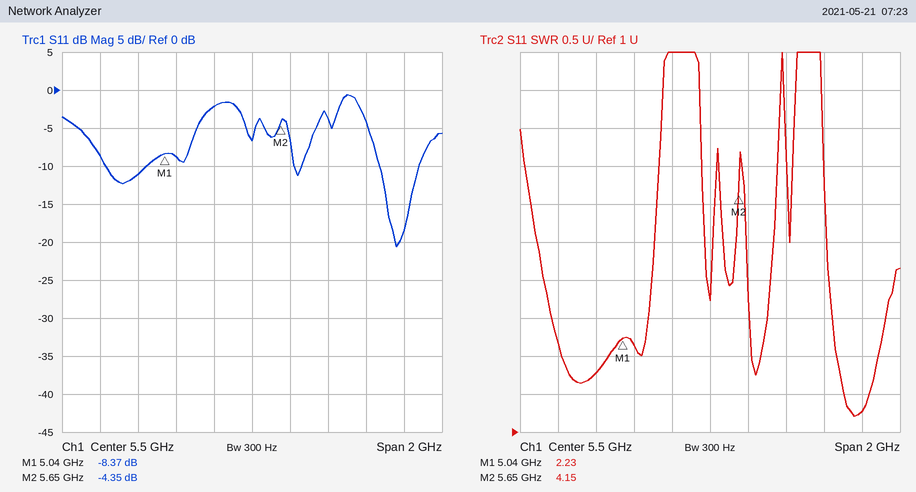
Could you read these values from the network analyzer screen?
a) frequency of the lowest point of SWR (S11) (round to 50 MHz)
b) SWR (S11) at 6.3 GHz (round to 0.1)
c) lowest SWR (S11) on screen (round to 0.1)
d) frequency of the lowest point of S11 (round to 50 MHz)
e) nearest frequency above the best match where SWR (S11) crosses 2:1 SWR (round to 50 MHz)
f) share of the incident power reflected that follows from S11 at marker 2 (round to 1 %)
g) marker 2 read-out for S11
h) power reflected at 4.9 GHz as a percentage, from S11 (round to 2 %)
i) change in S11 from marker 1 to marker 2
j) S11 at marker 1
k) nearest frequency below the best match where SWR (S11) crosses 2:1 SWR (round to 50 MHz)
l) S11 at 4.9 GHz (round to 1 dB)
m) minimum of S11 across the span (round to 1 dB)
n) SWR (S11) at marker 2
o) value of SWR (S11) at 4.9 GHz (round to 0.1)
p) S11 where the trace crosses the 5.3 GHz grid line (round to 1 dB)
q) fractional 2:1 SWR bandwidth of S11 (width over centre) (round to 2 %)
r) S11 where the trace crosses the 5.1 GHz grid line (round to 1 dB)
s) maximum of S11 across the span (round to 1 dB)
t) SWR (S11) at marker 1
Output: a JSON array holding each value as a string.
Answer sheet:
["6.25 GHz", "1.3", "1.2", "6.25 GHz", "6.40 GHz", "37 %", "-4.35 dB", "8 %", "4.02 dB", "-8.37 dB", "6.15 GHz", "-11 dB", "-21 dB", "4.15", "1.8", "-2 dB", "4 %", "-9 dB", "-1 dB", "2.23"]
